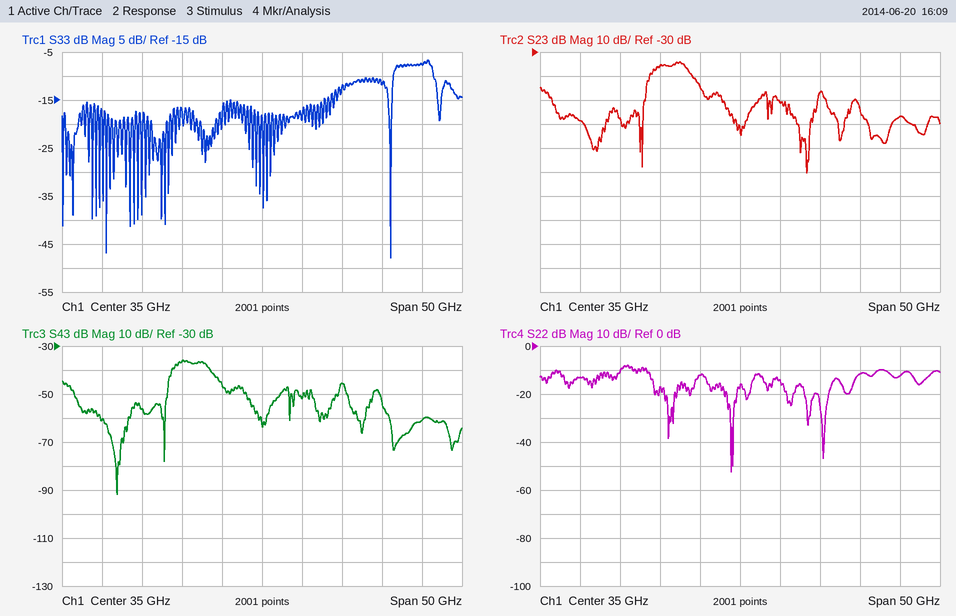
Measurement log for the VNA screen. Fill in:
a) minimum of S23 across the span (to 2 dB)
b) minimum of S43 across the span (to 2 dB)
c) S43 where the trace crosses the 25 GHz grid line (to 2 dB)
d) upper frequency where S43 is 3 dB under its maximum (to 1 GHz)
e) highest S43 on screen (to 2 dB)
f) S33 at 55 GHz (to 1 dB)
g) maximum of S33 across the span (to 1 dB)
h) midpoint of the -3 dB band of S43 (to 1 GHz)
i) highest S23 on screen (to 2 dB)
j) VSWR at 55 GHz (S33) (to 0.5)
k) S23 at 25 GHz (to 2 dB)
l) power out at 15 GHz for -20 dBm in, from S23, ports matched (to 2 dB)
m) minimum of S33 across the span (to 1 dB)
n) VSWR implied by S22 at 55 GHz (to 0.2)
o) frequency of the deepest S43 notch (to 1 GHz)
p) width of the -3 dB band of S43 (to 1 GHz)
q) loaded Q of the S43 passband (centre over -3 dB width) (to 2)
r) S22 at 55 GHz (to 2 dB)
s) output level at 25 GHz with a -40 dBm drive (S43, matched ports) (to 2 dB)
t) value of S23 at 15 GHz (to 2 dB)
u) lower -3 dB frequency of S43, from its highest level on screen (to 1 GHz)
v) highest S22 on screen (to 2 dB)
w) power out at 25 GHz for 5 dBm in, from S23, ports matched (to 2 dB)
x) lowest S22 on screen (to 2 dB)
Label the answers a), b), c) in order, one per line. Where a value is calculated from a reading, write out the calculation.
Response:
a) -80 dB
b) -92 dB
c) -36 dB
d) 28 GHz
e) -36 dB
f) -8 dB
g) -7 dB
h) 26 GHz
i) -34 dB
j) |Γ| = 10^(-8/20) = 0.3981; VSWR = (1 + 0.3981)/(1 − 0.3981) ≈ 2.32, so 2.5 to the nearest 0.5
k) -36 dB
l) -20 dBm + (-58 dB) = -78 dBm
m) -48 dB
n) |Γ| = 10^(-12/20) = 0.2512; VSWR = (1 + 0.2512)/(1 − 0.2512) ≈ 1.67, so 1.6 to the nearest 0.2
o) 17 GHz
p) 28 GHz − 24 GHz = 4 GHz
q) 26 GHz / 4 GHz ≈ 6
r) -12 dB
s) -40 dBm + (-36 dB) = -76 dBm
t) -58 dB
u) 24 GHz
v) -8 dB
w) 5 dBm + (-36 dB) = -30 dBm
x) -52 dB
